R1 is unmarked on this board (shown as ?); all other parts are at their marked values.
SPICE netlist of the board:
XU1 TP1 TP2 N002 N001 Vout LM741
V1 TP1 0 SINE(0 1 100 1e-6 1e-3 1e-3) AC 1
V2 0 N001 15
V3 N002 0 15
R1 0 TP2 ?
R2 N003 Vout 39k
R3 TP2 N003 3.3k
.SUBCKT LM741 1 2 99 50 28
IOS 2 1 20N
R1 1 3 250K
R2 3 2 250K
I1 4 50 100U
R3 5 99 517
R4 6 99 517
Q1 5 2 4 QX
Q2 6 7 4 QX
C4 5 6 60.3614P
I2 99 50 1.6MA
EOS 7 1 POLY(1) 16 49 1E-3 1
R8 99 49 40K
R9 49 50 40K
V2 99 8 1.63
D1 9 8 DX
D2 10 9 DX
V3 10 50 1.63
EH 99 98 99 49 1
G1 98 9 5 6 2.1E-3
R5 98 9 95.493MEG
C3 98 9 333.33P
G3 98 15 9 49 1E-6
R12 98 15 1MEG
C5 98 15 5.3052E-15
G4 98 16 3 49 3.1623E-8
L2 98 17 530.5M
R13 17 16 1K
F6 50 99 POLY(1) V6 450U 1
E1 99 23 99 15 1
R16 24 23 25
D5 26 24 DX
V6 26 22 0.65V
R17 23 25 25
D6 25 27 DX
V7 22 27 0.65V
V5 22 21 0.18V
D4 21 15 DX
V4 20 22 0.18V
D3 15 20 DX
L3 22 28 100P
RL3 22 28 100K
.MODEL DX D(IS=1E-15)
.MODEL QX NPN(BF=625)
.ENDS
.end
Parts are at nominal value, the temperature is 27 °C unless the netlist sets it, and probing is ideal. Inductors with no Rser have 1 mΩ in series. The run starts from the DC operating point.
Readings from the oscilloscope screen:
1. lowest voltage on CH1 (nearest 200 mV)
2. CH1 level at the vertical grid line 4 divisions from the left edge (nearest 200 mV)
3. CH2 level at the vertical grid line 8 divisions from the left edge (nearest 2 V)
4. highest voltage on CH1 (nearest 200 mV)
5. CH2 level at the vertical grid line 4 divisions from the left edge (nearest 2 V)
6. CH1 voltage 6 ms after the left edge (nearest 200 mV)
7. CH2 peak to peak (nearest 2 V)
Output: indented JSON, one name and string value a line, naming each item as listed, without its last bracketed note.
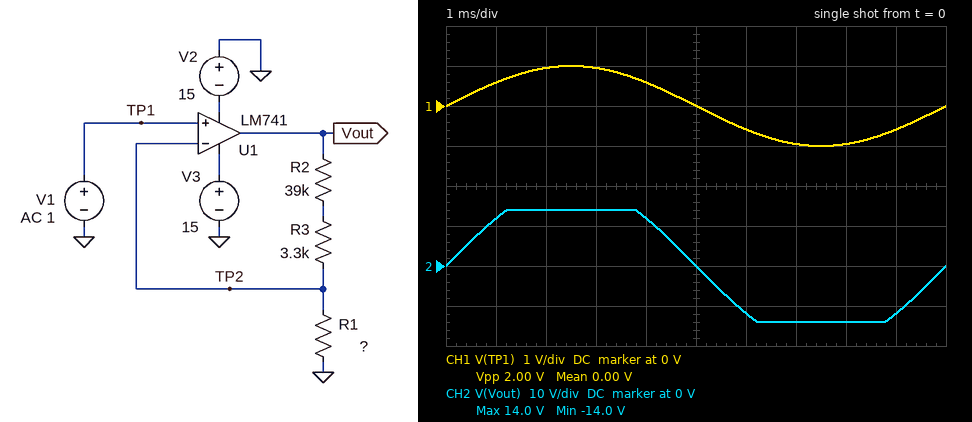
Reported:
{
  "lowest voltage on CH1": "-1.0 V",
  "CH1 level at the vertical grid line 4 divisions from the left edge": "600 mV",
  "CH2 level at the vertical grid line 8 divisions from the left edge": "-14 V",
  "highest voltage on CH1": "1.0 V",
  "CH2 level at the vertical grid line 4 divisions from the left edge": "12 V",
  "CH1 voltage 6 ms after the left edge": "-600 mV",
  "CH2 peak to peak": "28 V"
}
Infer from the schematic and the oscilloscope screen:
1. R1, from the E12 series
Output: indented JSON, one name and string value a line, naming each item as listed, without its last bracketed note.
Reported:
{
  "R1, from the E12 series": "2.2 kΩ"
}
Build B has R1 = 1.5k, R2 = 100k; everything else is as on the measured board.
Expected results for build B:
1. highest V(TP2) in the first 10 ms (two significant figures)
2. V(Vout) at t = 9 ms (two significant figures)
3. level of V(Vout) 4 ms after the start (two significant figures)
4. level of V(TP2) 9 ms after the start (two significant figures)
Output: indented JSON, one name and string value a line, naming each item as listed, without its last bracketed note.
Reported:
{
  "highest V(TP2) in the first 10 ms": "200 mV",
  "V(Vout) at t = 9 ms": "-14 V",
  "level of V(Vout) 4 ms after the start": "14 V",
  "level of V(TP2) 9 ms after the start": "-200 mV"
}
